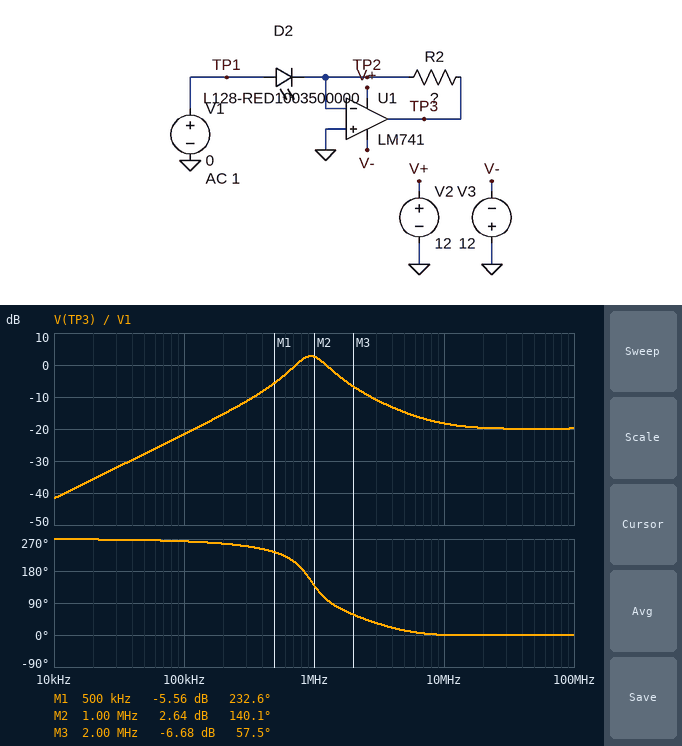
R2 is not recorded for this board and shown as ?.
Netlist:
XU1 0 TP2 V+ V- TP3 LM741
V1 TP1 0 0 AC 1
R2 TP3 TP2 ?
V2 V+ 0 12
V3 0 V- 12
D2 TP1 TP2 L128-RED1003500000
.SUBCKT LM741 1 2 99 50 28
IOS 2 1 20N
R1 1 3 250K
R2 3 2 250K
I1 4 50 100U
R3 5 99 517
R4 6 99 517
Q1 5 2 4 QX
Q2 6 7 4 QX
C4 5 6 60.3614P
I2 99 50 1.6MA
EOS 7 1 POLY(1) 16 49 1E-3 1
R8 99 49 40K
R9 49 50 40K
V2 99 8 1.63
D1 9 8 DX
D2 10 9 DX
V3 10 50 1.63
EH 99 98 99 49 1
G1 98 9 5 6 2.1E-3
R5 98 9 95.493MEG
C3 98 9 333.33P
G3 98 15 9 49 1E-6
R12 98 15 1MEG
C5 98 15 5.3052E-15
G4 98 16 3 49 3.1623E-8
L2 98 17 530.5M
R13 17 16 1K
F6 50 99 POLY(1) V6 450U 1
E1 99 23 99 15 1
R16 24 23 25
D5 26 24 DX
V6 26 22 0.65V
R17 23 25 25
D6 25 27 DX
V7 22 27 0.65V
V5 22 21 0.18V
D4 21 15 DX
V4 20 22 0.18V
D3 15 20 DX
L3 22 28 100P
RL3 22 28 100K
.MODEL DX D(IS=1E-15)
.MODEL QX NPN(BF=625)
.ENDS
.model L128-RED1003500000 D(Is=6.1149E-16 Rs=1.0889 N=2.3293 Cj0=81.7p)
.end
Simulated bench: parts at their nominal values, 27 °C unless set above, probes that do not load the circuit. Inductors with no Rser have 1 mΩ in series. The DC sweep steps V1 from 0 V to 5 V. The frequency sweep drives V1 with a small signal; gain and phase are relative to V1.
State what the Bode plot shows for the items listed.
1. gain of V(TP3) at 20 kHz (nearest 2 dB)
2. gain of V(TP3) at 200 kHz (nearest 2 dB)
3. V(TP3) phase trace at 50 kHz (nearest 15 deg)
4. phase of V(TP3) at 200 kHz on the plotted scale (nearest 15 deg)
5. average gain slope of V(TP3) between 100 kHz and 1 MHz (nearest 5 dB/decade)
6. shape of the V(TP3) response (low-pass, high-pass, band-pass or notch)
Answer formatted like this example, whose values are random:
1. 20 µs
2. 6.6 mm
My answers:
1. -36 dB
2. -16 dB
3. 270 deg
4. 255 deg
5. 25 dB/decade
6. band-pass
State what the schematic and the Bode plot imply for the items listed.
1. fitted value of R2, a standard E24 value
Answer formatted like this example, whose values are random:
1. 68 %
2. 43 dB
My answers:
1. 1.6 kΩ
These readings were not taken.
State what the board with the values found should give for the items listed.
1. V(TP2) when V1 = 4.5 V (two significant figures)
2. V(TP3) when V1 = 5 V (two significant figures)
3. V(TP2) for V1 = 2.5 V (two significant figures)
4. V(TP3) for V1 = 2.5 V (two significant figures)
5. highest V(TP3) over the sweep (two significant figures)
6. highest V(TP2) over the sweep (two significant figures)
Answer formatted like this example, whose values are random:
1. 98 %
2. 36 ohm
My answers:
1. 2.7 V
2. -11 V
3. 680 mV
4. -11 V
5. 1.2 mV
6. 3.2 V
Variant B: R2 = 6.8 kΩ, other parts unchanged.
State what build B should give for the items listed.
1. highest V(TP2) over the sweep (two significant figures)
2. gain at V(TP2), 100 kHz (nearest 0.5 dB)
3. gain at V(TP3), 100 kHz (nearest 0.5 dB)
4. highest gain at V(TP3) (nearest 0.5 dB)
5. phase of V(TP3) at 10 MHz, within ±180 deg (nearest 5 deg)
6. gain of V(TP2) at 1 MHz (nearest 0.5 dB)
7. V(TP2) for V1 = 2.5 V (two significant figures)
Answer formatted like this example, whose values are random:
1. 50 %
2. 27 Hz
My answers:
1. 3.3 V
2. -28.5 dB
3. -9.0 dB
4. 15.5 dB
5. -15 deg
6. 2.0 dB
7. 770 mV
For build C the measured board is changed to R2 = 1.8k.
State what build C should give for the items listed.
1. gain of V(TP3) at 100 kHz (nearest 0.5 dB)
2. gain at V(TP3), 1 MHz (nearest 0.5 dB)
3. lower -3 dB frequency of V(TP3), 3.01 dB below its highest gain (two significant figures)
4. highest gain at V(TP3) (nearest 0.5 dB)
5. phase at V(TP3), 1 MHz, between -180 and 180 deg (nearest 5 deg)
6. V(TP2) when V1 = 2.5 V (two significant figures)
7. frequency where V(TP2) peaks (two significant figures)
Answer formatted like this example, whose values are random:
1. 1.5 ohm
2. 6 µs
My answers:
1. -20.5 dB
2. 3.5 dB
3. 690 kHz
4. 4.0 dB
5. 130 deg
6. 690 mV
7. 980 kHz
